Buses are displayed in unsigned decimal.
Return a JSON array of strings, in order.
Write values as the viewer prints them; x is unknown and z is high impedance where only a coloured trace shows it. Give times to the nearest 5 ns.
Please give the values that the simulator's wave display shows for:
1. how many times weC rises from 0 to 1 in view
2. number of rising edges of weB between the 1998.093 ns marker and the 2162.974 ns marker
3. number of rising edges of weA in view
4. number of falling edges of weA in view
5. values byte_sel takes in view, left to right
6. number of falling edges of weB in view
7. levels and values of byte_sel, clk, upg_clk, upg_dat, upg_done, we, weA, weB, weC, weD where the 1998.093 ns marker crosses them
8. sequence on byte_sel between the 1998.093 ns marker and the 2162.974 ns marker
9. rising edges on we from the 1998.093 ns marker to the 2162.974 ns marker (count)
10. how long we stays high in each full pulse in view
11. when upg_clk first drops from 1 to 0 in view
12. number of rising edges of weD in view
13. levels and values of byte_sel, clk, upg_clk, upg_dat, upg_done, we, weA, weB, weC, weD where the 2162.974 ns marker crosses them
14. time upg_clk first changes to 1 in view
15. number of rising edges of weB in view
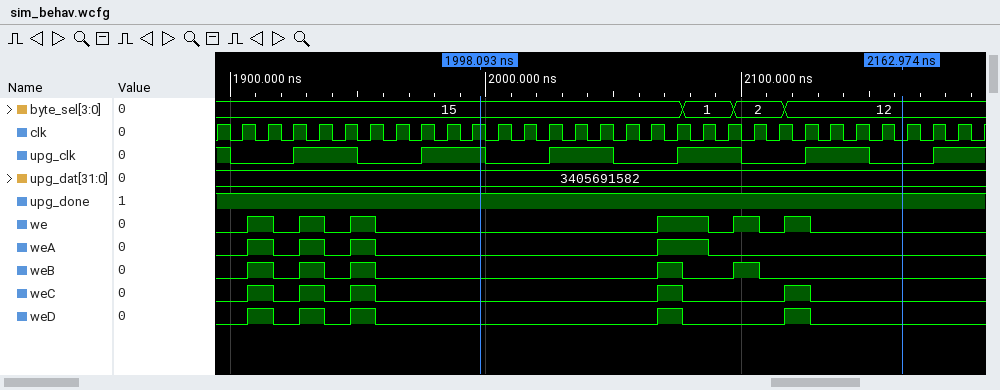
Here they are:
["5", "2", "4", "4", "15, 1, 2, 12", "5", "byte_sel=15, clk=1, upg_clk=1, upg_dat=3405691582, upg_done=1, we=0, weA=0, weB=0, weC=0, weD=0", "15, 1, 2, 12", "3", "10 ns, 10 ns, 10 ns, 20 ns, 10 ns, 10 ns", "1900 ns", "5", "byte_sel=12, clk=0, upg_clk=0, upg_dat=3405691582, upg_done=1, we=0, weA=0, weB=0, weC=0, weD=0", "1925 ns", "5"]
